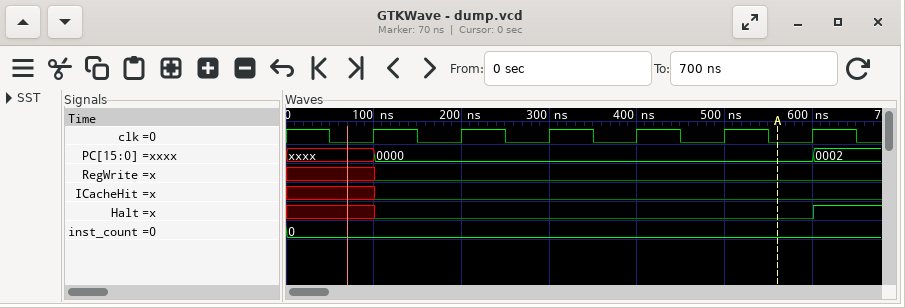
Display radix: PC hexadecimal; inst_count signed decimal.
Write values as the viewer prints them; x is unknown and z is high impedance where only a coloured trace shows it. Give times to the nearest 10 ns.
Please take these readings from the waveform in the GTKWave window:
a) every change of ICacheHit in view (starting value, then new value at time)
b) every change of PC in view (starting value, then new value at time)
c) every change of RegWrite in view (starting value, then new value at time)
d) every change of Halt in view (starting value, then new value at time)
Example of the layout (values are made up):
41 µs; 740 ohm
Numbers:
x, 0 at 100 ns; xxxx, 0000 at 100 ns, 0002 at 600 ns; x, 0 at 100 ns; x, 0 at 100 ns, 1 at 600 ns
